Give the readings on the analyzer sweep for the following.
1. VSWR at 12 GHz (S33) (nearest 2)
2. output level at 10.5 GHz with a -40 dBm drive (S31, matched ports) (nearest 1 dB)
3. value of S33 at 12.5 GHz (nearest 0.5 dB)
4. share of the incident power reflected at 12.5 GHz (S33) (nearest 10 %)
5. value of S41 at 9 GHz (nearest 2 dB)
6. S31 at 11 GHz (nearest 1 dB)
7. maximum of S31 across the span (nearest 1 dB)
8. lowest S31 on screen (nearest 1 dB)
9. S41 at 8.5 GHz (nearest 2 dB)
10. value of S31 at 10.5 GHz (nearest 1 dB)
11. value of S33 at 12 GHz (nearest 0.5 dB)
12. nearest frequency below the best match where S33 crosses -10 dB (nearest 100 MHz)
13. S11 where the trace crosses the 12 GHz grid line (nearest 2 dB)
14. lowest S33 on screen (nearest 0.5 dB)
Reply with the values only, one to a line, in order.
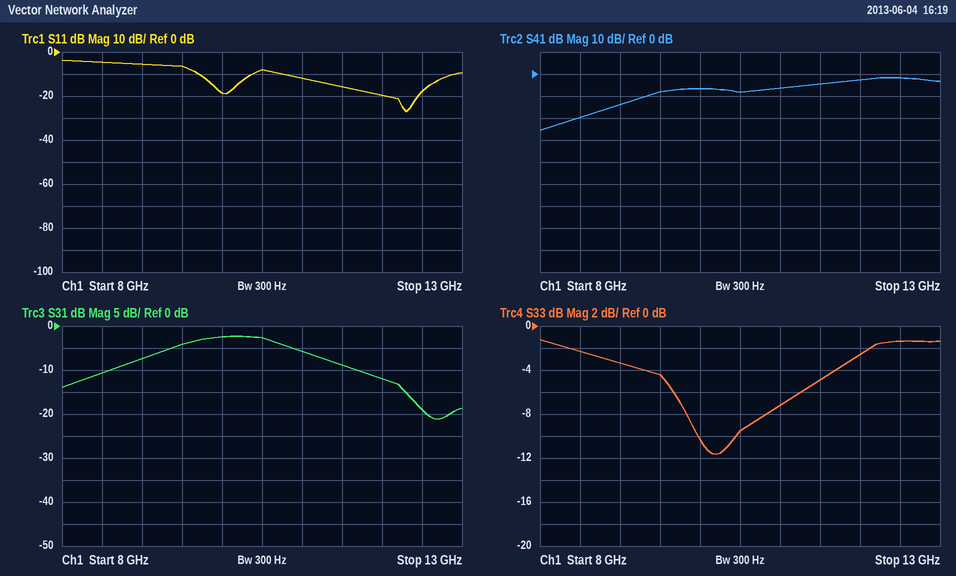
6
-43 dBm
-1.5 dB
70 %
-14 dB
-6 dB
-2 dB
-21 dB
-20 dB
-3 dB
-2.5 dB
10.0 GHz
-20 dB
-11.5 dB
